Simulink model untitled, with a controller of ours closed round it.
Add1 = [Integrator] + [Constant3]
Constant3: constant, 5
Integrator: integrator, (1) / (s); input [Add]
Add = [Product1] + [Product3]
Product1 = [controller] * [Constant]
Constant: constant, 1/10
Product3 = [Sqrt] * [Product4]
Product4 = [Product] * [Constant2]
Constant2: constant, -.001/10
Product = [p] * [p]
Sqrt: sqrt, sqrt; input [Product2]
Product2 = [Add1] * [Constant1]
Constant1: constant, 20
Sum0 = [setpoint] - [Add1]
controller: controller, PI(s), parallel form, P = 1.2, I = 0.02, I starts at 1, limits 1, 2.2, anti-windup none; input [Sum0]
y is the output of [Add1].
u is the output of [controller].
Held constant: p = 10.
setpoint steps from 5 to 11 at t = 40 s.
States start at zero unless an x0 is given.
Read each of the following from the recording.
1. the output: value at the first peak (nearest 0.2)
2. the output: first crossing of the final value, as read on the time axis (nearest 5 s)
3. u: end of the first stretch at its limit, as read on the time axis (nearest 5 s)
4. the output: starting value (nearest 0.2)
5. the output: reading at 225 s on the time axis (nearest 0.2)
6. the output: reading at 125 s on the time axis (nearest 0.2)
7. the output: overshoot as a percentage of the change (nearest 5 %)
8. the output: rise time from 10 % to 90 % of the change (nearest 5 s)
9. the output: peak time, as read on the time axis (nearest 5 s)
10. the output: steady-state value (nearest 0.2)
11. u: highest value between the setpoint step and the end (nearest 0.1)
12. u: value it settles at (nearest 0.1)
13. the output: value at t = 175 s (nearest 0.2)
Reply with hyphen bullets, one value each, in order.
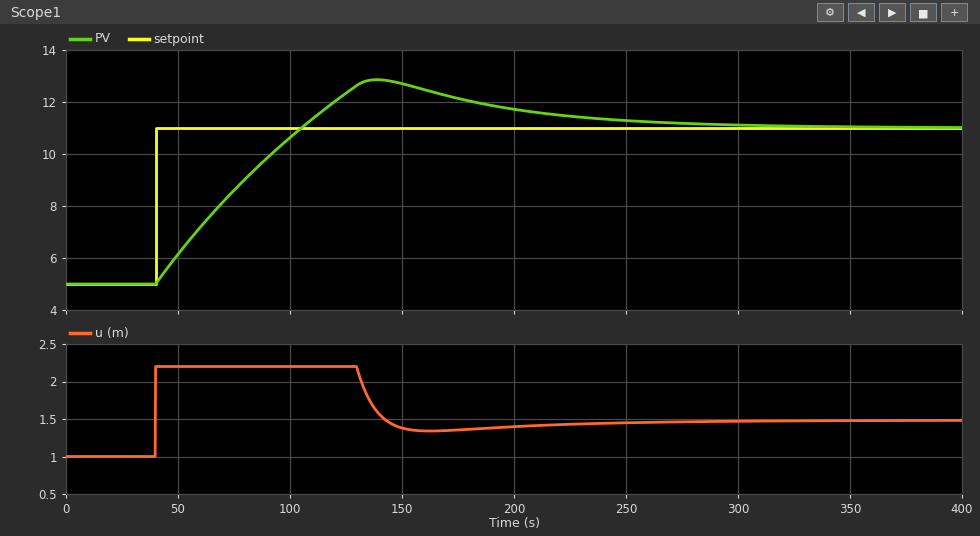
- 12.8
- 105 s
- 130 s
- 5.0
- 11.4
- 12.4
- 30 %
- 50 s
- 140 s
- 11.0
- 2.2
- 1.5
- 12.2
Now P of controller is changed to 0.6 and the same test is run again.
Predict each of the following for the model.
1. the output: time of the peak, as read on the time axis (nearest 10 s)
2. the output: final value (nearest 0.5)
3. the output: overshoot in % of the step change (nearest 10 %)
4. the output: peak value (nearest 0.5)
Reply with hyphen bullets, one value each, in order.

- 150 s
- 11.0
- 40 %
- 13.5
